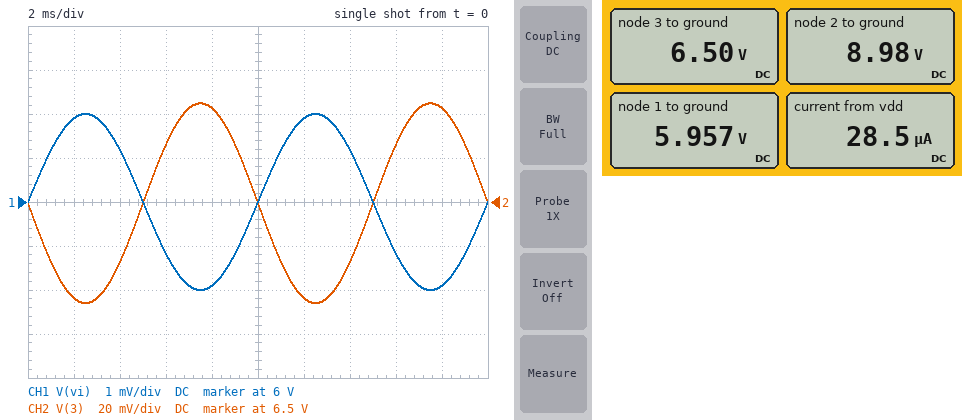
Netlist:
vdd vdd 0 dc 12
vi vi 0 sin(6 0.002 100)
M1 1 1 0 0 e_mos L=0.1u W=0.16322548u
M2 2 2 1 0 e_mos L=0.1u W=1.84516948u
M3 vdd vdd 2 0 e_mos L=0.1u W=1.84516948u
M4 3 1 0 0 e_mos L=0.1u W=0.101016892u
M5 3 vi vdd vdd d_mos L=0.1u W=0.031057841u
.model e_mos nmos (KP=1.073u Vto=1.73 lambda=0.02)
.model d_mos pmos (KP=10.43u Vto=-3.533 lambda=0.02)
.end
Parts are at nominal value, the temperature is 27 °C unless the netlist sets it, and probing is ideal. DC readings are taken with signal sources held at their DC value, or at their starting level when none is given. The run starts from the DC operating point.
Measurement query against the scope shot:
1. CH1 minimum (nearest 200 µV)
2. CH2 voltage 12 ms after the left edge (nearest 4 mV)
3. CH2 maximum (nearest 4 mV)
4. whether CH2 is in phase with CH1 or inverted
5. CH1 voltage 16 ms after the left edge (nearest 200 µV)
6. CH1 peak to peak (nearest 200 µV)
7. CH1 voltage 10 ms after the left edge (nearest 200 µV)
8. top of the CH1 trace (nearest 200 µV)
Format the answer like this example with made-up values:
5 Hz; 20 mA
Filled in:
5.9980 V; 6.456 V; 6.544 V; inverted; 5.9988 V; 4.0 mV; 6.0000 V; 6.0020 V
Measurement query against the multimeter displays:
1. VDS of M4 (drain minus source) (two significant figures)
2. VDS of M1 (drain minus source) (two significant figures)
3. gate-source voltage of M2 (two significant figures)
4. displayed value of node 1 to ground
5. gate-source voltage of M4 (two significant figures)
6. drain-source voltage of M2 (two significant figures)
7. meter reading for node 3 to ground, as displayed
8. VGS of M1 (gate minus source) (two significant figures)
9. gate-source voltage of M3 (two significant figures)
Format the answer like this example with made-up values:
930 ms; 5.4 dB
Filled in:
6.5 V; 6.0 V; 3.0 V; 5.957 V; 6.0 V; 3.0 V; 6.50 V; 6.0 V; 3.0 V
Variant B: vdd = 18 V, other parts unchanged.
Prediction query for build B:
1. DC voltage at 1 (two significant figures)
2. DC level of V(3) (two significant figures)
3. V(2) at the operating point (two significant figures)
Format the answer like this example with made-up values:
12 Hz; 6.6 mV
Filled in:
9.6 V; 16 V; 14 V
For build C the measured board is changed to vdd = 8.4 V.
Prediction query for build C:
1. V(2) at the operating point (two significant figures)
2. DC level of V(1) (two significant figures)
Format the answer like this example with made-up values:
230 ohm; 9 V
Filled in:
6.1 V; 3.7 V
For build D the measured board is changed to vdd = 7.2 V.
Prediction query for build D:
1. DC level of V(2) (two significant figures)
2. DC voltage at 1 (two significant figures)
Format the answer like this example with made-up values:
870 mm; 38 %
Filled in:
5.1 V; 3.0 V
